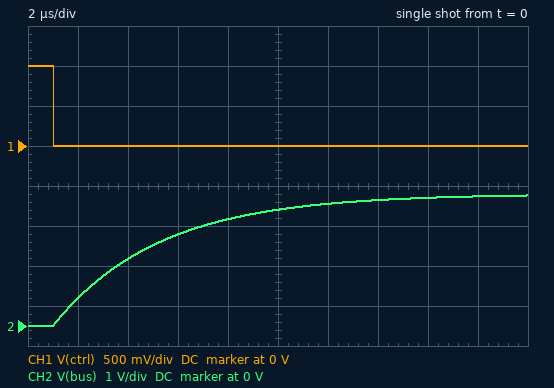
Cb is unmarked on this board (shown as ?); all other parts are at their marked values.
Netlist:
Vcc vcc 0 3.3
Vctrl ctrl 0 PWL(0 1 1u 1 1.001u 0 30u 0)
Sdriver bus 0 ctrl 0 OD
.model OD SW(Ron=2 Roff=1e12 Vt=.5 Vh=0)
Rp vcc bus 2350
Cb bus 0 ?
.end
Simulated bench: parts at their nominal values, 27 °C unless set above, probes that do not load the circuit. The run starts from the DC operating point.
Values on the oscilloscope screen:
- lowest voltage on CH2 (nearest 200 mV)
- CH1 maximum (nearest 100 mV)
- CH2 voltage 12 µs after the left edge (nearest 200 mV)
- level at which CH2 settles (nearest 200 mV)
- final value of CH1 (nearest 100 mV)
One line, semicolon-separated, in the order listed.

0 V; 1.0 V; 3.0 V; 3.2 V; 0 V
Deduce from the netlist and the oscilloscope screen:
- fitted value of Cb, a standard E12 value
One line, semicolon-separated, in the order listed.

1.8 nF
